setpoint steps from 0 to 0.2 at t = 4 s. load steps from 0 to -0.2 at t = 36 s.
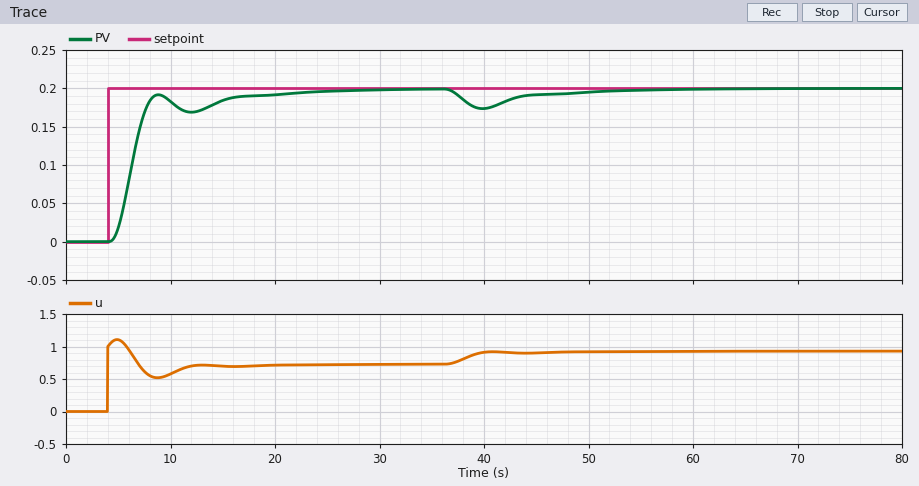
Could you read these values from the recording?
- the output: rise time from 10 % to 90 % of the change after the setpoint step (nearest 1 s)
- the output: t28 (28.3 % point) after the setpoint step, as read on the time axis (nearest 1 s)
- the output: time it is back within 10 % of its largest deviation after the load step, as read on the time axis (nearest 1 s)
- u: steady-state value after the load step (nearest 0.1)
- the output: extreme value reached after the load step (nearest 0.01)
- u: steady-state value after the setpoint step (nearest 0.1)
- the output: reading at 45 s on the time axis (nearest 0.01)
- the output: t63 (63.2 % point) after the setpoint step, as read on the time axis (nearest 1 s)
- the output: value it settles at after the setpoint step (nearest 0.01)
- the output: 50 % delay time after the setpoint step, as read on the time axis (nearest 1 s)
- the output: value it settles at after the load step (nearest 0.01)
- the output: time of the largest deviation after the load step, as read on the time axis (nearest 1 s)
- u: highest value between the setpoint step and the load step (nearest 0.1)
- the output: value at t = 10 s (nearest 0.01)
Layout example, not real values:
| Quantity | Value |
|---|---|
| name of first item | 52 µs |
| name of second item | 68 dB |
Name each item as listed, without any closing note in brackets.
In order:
| Quantity | Value |
|---|---|
| the output: rise time from 10 % to 90 % of the change after the setpoint step | 3 s |
| the output: t28 (28.3 % point) after the setpoint step, as read on the time axis | 6 s |
| the output: time it is back within 10 % of its largest deviation after the load step, as read on the time axis | 55 s |
| u: steady-state value after the load step | 0.9 |
| the output: extreme value reached after the load step | 0.17 |
| u: steady-state value after the setpoint step | 0.7 |
| the output: reading at 45 s on the time axis | 0.19 |
| the output: t63 (63.2 % point) after the setpoint step, as read on the time axis | 7 s |
| the output: value it settles at after the setpoint step | 0.20 |
| the output: 50 % delay time after the setpoint step, as read on the time axis | 6 s |
| the output: value it settles at after the load step | 0.20 |
| the output: time of the largest deviation after the load step, as read on the time axis | 40 s |
| u: highest value between the setpoint step and the load step | 1.1 |
| the output: value at t = 10 s | 0.18 |
